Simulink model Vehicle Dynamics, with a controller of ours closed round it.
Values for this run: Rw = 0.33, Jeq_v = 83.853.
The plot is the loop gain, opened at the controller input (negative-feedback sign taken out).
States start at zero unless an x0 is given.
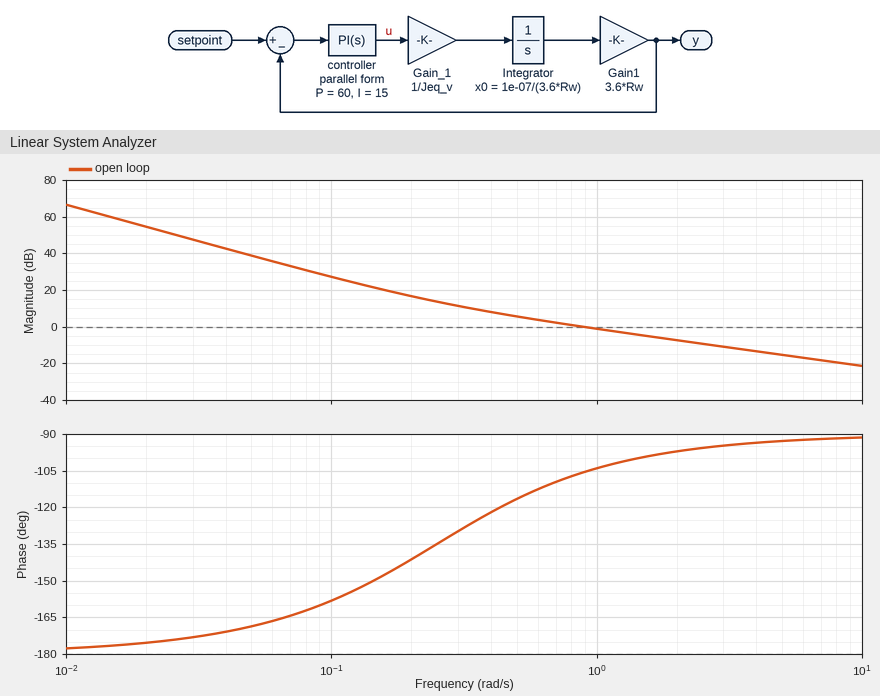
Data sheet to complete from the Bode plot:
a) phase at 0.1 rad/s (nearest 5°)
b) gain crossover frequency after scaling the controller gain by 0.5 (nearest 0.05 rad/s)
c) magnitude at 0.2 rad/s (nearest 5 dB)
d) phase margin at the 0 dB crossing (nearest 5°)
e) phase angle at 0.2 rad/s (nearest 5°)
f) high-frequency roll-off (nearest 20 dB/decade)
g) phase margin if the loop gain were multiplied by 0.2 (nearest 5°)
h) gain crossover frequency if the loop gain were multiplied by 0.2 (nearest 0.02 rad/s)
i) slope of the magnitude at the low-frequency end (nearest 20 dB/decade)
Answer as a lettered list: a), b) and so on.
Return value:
a) -160°
b) 0.50 rad/s
c) 15 dB
d) 75°
e) -140°
f) -20 dB/decade
g) 45°
h) 0.24 rad/s
i) -40 dB/decade
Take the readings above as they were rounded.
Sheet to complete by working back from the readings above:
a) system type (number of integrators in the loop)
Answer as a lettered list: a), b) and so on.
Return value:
a) 2
